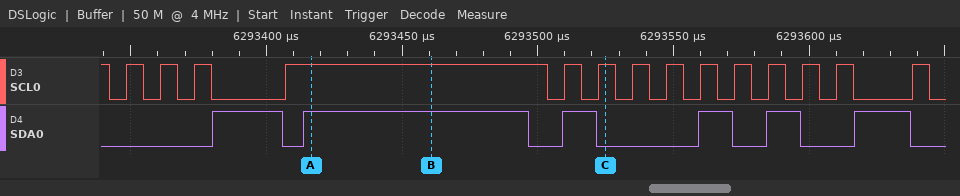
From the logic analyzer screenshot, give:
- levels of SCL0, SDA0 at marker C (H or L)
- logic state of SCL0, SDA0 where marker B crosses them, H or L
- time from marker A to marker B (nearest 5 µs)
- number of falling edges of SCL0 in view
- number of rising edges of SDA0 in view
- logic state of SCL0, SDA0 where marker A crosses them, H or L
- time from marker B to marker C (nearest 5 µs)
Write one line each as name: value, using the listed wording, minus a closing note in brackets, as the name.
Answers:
levels of SCL0, SDA0 at marker C: SCL0=H, SDA0=L
logic state of SCL0, SDA0 where marker B crosses them, H or L: SCL0=H, SDA0=H
time from marker A to marker B: 45 µs
number of falling edges of SCL0 in view: 15
number of rising edges of SDA0 in view: 6
logic state of SCL0, SDA0 where marker A crosses them, H or L: SCL0=H, SDA0=H
time from marker B to marker C: 65 µs
